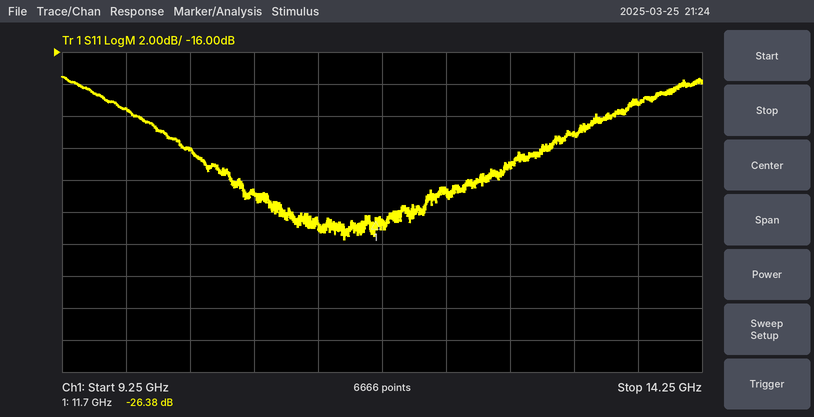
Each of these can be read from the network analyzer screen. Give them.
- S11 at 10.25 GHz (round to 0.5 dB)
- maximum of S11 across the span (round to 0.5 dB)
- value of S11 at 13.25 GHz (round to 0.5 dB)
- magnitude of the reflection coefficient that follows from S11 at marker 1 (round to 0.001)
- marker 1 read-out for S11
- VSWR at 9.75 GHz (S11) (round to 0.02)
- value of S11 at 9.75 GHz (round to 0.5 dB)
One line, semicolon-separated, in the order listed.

-22.0 dB; -17.5 dB; -21.0 dB; 0.048; -26.38 dB; 1.24; -19.5 dB
